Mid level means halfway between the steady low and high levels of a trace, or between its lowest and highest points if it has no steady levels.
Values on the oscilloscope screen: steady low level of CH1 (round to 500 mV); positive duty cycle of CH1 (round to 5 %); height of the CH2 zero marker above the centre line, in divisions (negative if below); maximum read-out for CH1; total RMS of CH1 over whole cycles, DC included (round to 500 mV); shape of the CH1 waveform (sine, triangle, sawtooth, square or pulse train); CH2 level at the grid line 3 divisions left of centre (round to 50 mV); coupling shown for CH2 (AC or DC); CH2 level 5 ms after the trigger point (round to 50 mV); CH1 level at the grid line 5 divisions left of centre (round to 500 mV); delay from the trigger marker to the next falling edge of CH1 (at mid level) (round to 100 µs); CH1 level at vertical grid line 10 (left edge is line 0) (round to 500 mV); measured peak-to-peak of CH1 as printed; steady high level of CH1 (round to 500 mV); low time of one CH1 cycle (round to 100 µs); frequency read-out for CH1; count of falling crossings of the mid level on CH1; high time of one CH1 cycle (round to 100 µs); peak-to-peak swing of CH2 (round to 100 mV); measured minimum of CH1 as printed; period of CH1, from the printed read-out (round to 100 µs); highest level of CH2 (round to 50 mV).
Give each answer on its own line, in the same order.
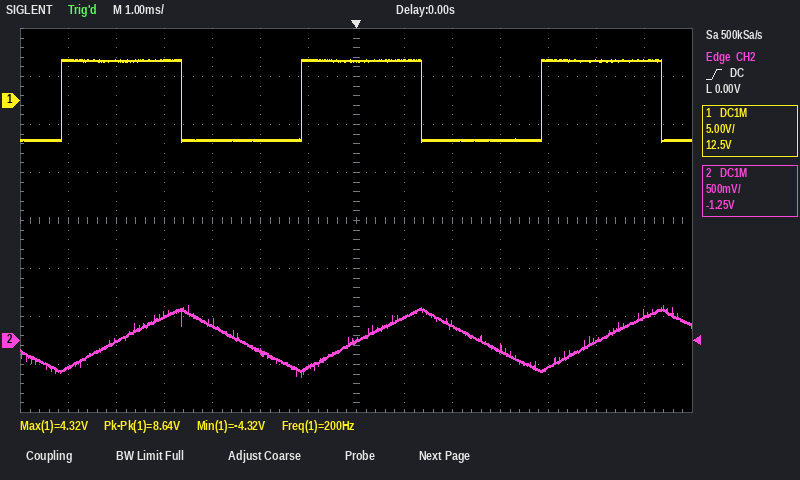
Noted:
-4.0 V
50 %
-2.5 div
4.32 V
4.0 V
square
200 mV
DC
0 mV
4.0 V
1.4 ms
-4.0 V
8.64 V
4.0 V
2.5 ms
200 Hz
3
2.5 ms
700 mV
-4.32 V
5.0 ms
350 mV
